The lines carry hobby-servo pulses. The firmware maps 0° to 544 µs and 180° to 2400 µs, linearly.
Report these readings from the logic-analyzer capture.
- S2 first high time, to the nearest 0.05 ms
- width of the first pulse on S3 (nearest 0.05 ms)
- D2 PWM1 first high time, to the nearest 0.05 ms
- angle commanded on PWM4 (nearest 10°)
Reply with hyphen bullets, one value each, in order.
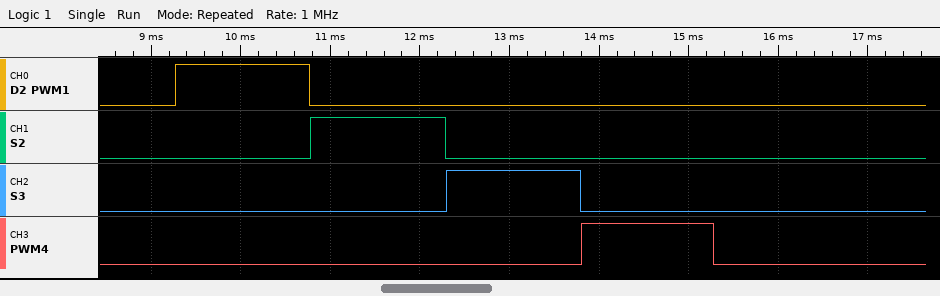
- 1.50 ms
- 1.50 ms
- 1.50 ms
- 90°
